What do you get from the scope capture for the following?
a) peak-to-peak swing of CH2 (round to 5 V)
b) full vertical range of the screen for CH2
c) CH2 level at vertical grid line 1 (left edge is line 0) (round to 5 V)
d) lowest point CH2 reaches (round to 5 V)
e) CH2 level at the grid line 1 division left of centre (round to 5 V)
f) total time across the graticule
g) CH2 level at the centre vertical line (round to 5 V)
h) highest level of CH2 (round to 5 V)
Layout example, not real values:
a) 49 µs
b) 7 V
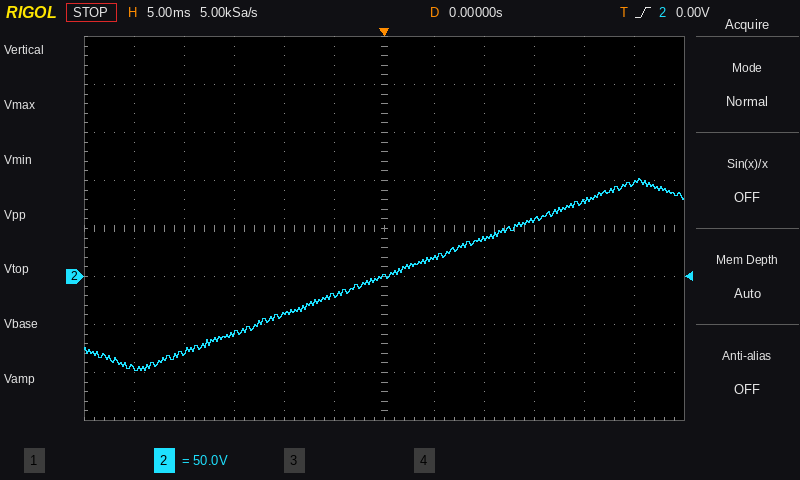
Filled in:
a) 200 V
b) 400 V
c) -95 V
d) -100 V
e) -20 V
f) 60 ms
g) 0 V
h) 100 V
